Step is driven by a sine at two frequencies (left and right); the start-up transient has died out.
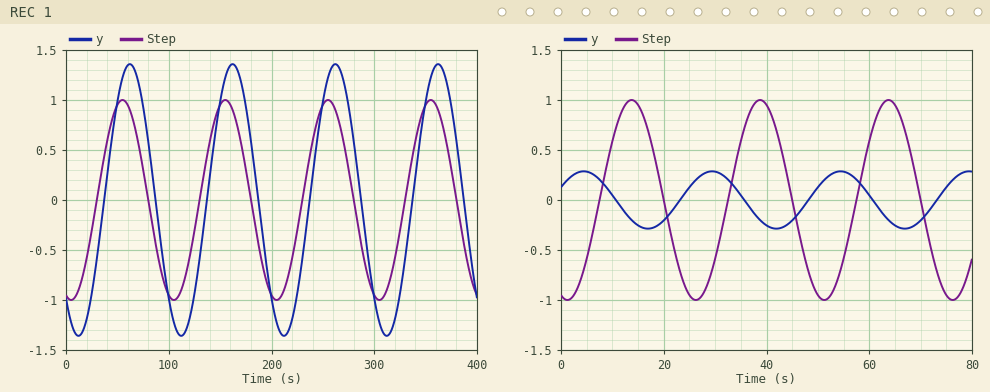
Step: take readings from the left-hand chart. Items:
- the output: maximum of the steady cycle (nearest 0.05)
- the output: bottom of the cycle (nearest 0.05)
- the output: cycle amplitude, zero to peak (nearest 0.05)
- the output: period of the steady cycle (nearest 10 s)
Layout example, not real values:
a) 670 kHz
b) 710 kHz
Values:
a) 1.35
b) -1.35
c) 1.35
d) 100 s
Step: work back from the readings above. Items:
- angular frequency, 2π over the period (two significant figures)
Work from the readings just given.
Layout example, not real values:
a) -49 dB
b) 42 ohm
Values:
a) 0.063 rad/s
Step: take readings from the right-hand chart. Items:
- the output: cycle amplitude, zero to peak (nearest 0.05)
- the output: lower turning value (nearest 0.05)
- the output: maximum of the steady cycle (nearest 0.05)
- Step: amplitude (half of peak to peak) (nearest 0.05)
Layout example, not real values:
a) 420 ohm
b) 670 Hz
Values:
a) 0.30
b) -0.30
c) 0.30
d) 1.00
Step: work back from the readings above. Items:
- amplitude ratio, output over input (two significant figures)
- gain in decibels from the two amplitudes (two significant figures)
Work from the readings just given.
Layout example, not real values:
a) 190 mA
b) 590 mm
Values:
a) 0.30
b) -10 dB
